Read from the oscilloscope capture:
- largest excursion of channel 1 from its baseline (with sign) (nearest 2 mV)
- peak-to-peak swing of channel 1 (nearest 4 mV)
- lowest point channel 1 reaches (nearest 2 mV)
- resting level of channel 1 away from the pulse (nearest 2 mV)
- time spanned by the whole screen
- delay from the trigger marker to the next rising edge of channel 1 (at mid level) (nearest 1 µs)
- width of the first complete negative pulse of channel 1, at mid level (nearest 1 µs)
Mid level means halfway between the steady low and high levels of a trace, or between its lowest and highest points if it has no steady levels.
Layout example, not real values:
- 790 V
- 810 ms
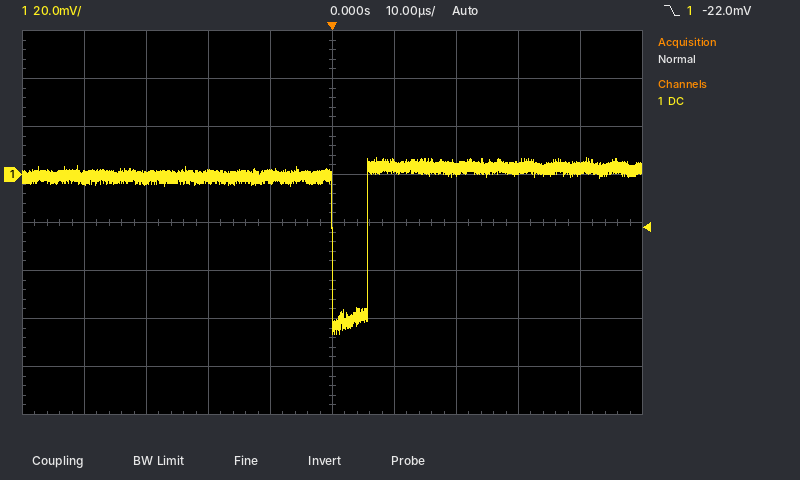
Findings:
- -66 mV
- 72 mV
- -66 mV
- 0 mV
- 100 µs
- 6 µs
- 6 µs
